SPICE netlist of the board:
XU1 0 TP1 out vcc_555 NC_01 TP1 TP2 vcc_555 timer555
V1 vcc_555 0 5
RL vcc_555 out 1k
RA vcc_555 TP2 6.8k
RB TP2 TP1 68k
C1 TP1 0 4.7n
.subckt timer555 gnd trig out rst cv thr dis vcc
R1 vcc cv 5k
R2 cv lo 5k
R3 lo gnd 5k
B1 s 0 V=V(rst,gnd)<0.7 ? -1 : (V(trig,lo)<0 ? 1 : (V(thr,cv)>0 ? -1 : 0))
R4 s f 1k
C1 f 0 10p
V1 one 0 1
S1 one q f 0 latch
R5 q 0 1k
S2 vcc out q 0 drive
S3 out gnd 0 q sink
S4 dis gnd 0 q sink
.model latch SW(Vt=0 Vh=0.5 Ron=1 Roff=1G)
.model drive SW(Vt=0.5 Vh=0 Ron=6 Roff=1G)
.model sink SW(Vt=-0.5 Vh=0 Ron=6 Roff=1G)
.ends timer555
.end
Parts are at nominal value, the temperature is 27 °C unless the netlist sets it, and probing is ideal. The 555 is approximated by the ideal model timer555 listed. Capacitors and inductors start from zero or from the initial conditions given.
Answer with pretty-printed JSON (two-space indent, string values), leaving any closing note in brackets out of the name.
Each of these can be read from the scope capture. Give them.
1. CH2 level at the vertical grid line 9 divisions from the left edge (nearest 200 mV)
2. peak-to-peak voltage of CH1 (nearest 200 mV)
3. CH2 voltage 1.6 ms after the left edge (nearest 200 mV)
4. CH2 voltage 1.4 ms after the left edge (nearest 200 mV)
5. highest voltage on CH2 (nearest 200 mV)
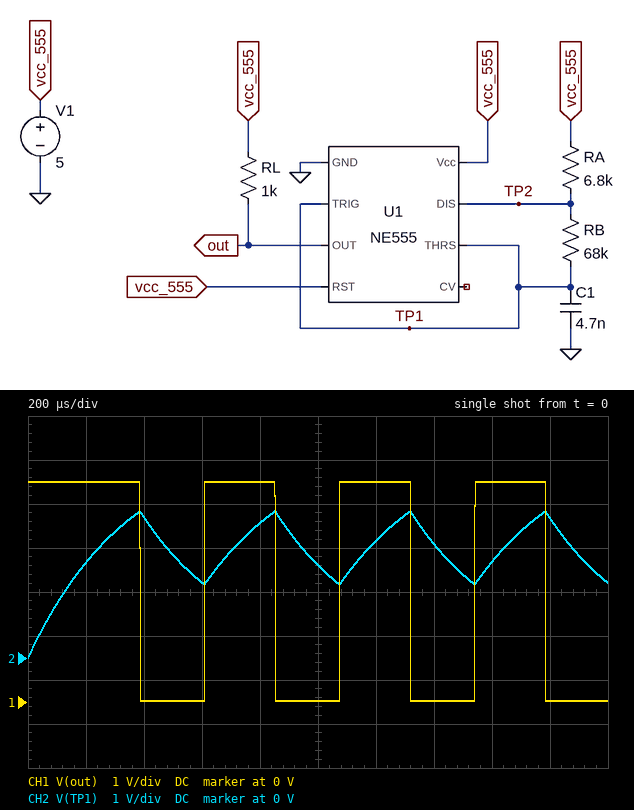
{
  "CH2 level at the vertical grid line 9 divisions from the left edge": "3.2 V",
  "peak-to-peak voltage of CH1": "5.0 V",
  "CH2 voltage 1.6 ms after the left edge": "2.2 V",
  "CH2 voltage 1.4 ms after the left edge": "2.6 V",
  "highest voltage on CH2": "3.4 V"
}
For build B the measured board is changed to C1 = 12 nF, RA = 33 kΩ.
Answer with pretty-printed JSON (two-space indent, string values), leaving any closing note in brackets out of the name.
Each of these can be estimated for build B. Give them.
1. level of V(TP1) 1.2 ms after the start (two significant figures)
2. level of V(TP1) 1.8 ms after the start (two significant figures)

{
  "level of V(TP1) 1.2 ms after the start": "3.1 V",
  "level of V(TP1) 1.8 ms after the start": "1.9 V"
}
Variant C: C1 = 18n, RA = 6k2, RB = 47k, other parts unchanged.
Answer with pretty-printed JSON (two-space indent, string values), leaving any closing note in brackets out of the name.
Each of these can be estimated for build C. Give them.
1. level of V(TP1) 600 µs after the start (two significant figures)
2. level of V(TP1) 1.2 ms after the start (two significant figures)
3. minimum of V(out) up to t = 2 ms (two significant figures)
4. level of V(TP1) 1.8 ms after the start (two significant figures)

{
  "level of V(TP1) 600 µs after the start": "2.3 V",
  "level of V(TP1) 1.2 ms after the start": "2.8 V",
  "minimum of V(out) up to t = 2 ms": "30 mV",
  "level of V(TP1) 1.8 ms after the start": "2.2 V"
}
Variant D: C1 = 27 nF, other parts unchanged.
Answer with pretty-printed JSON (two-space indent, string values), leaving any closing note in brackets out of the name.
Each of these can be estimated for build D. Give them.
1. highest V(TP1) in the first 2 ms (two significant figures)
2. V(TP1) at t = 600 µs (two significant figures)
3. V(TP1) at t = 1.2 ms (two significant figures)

{
  "highest V(TP1) in the first 2 ms": "3.1 V",
  "V(TP1) at t = 600 µs": "1.3 V",
  "V(TP1) at t = 1.2 ms": "2.2 V"
}
